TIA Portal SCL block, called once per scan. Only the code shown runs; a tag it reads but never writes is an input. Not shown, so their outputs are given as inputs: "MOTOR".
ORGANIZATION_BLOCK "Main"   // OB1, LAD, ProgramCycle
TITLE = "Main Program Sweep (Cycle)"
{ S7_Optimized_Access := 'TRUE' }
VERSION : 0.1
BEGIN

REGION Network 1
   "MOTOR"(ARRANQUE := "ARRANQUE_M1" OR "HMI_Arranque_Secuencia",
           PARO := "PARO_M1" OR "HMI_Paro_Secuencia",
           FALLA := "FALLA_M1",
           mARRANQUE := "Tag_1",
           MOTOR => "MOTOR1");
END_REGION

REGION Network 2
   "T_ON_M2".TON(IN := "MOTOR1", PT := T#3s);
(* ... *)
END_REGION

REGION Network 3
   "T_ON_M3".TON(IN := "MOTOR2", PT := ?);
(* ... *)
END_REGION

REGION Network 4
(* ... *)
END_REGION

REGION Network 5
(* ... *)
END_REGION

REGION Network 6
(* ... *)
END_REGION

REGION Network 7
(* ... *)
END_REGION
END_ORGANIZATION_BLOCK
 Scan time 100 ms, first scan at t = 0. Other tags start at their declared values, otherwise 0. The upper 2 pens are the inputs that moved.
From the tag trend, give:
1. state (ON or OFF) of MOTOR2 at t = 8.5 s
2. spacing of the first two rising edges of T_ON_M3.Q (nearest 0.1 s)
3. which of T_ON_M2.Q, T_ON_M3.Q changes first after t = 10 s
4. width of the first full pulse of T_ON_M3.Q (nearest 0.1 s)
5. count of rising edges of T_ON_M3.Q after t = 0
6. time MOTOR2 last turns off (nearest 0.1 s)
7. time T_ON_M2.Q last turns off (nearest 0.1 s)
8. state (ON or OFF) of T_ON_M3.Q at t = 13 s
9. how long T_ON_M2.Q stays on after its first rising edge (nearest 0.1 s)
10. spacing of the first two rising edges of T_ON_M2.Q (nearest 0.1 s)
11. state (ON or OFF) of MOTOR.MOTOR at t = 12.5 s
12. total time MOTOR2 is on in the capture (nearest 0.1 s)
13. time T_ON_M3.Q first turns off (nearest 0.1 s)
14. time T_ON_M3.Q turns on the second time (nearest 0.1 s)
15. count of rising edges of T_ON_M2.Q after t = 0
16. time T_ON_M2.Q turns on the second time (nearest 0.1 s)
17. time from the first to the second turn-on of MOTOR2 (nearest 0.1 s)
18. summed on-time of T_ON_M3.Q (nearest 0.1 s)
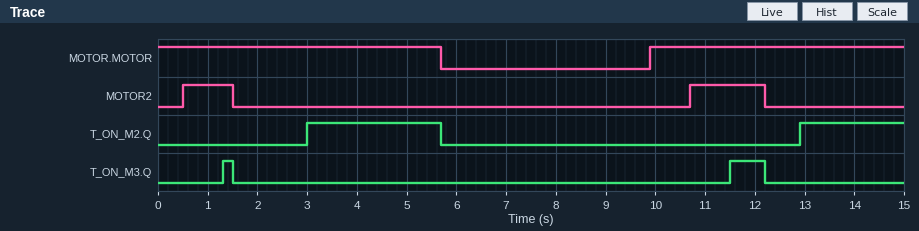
OFF
10.2 s
T_ON_M3.Q
0.2 s
2
12.2 s
5.7 s
OFF
2.7 s
9.9 s
ON
2.5 s
1.5 s
11.5 s
2
12.9 s
10.2 s
0.9 s
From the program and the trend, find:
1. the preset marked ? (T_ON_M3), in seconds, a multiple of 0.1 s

0.8 s
